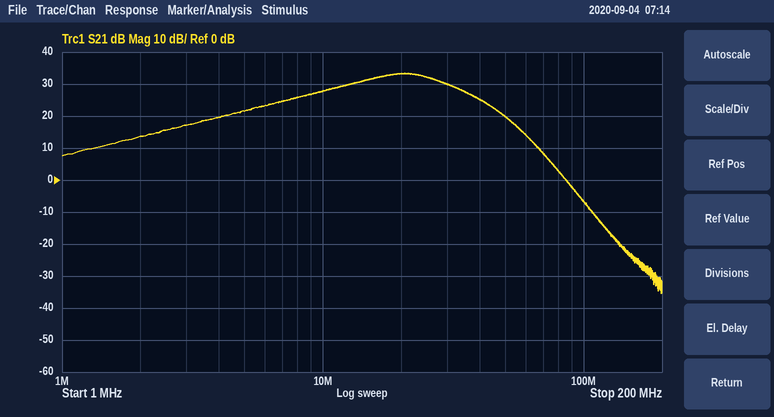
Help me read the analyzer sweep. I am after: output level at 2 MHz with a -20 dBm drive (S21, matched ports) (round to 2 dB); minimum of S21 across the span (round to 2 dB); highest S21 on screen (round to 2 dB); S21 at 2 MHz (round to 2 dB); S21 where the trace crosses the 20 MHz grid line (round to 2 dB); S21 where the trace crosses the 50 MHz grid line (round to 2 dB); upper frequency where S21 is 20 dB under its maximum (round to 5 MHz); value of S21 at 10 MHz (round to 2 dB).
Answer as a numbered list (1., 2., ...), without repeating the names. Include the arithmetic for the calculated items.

1. -20 dBm + (14 dB) = -6 dBm
2. -36 dB
3. 34 dB
4. 14 dB
5. 34 dB
6. 20 dB
7. 60 MHz
8. 28 dB
